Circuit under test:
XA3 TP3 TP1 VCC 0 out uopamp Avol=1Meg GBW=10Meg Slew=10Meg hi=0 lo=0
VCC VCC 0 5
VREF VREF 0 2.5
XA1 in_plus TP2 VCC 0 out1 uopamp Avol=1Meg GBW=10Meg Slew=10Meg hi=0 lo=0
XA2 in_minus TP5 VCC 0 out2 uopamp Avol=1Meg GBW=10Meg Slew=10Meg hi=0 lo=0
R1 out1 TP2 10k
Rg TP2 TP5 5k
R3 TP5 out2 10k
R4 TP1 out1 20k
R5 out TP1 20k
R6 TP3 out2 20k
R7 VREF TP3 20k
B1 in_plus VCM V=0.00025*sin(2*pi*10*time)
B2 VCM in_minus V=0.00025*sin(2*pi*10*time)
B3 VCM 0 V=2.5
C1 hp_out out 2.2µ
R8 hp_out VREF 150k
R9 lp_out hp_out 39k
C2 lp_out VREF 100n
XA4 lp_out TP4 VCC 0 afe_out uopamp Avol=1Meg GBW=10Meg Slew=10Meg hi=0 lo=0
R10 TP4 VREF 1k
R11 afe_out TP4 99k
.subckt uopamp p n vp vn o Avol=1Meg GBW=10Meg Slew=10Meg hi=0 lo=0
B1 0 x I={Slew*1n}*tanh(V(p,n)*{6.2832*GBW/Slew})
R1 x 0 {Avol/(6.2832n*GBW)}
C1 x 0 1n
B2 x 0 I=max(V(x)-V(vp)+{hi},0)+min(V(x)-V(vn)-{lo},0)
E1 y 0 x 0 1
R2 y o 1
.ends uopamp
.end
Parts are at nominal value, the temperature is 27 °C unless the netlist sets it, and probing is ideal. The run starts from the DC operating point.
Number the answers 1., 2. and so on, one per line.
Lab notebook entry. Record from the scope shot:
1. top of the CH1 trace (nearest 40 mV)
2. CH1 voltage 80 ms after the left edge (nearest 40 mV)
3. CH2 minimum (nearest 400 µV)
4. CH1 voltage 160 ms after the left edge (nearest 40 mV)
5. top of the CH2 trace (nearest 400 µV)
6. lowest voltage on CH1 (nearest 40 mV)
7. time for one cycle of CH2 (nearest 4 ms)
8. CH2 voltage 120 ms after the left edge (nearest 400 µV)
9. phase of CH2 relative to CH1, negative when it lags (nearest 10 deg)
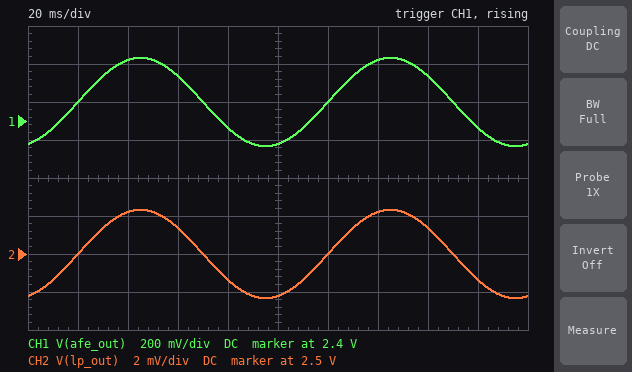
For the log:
1. 2.72 V
2. 2.36 V
3. 2.4976 V
4. 2.64 V
5. 2.5024 V
6. 2.28 V
7. 100 ms
8. 2.5000 V
9. 0 deg
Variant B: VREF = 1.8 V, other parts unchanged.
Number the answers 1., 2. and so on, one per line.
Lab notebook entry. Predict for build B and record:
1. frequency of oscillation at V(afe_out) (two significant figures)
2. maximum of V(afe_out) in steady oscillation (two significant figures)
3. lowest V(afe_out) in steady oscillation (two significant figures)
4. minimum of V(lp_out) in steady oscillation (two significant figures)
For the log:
1. 10 Hz
2. 2.0 V
3. 1.6 V
4. 1.8 V
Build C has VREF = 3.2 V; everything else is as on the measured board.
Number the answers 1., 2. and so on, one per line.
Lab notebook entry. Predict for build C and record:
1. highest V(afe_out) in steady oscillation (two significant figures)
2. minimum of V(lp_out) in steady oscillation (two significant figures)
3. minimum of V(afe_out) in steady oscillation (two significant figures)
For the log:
1. 3.4 V
2. 3.2 V
3. 3.0 V
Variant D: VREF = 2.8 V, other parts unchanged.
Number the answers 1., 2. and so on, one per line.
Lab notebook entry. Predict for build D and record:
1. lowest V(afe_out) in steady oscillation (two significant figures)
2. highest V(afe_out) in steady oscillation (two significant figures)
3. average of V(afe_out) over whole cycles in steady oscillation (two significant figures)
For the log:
1. 2.6 V
2. 3.0 V
3. 2.8 V
